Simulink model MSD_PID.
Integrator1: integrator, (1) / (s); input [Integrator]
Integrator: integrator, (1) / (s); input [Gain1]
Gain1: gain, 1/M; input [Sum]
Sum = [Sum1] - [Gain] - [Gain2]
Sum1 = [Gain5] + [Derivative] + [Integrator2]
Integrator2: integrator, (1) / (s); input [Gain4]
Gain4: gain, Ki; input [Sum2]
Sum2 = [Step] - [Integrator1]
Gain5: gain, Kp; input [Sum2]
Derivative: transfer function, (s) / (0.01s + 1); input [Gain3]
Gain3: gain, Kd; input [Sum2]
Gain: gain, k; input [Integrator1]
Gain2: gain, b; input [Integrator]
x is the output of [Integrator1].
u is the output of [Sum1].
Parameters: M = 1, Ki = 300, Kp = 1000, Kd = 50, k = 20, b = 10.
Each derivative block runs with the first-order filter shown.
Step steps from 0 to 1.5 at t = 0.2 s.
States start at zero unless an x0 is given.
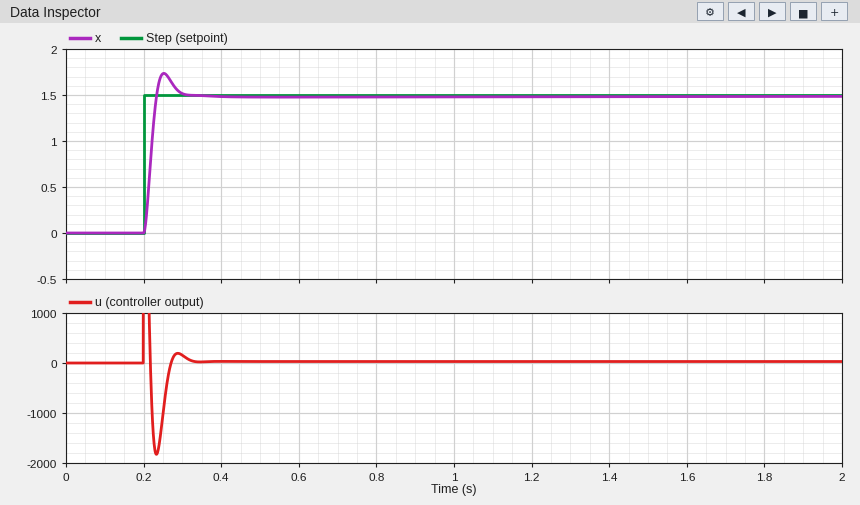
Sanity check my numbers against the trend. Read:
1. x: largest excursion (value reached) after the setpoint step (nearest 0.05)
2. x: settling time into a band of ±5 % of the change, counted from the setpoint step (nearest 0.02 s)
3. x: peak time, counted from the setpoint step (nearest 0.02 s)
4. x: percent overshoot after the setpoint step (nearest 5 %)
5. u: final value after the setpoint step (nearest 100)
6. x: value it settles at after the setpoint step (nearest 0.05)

1.75
0.08 s
0.06 s
15 %
0
1.50
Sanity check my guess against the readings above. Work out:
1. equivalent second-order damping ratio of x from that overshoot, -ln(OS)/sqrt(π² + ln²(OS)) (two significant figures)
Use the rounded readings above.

0.52
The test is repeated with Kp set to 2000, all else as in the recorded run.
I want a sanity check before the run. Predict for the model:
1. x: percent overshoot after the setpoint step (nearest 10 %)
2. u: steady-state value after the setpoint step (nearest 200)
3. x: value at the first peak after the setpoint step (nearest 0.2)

30 %
0
2.0
